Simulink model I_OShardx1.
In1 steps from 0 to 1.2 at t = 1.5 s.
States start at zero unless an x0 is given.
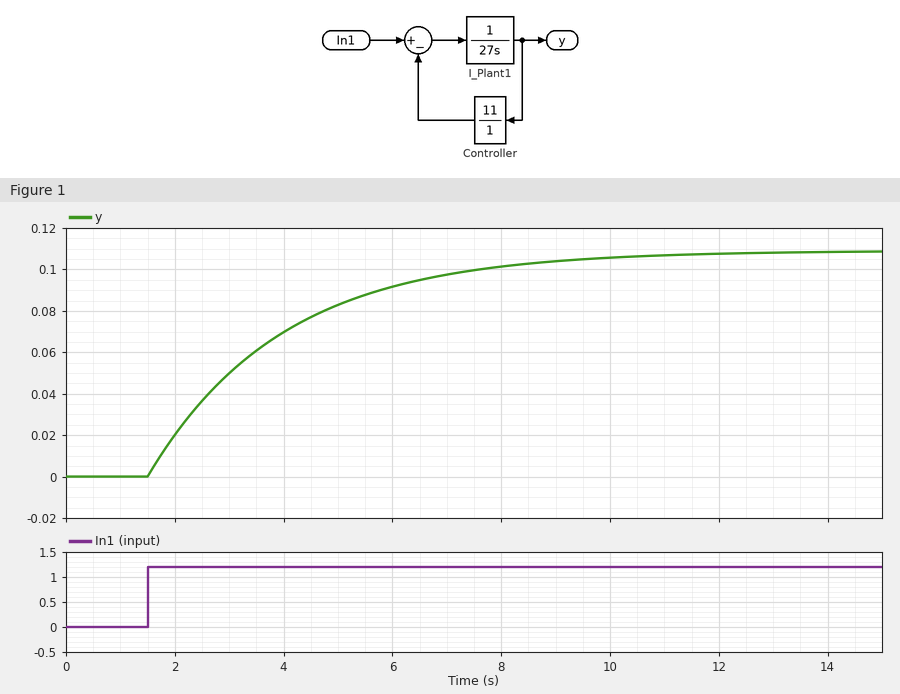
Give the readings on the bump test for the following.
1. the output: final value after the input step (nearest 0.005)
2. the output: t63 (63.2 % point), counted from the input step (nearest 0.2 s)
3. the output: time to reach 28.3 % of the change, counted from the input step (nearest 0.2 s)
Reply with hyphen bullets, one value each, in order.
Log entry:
- 0.110
- 2.4 s
- 0.8 s
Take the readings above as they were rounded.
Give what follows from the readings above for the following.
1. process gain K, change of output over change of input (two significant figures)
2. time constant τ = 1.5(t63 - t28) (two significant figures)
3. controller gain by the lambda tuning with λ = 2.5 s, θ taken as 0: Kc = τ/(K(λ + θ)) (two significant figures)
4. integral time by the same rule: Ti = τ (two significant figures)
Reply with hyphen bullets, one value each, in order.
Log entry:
- 0.092
- 2.4 s
- 10
- 2.4 s
